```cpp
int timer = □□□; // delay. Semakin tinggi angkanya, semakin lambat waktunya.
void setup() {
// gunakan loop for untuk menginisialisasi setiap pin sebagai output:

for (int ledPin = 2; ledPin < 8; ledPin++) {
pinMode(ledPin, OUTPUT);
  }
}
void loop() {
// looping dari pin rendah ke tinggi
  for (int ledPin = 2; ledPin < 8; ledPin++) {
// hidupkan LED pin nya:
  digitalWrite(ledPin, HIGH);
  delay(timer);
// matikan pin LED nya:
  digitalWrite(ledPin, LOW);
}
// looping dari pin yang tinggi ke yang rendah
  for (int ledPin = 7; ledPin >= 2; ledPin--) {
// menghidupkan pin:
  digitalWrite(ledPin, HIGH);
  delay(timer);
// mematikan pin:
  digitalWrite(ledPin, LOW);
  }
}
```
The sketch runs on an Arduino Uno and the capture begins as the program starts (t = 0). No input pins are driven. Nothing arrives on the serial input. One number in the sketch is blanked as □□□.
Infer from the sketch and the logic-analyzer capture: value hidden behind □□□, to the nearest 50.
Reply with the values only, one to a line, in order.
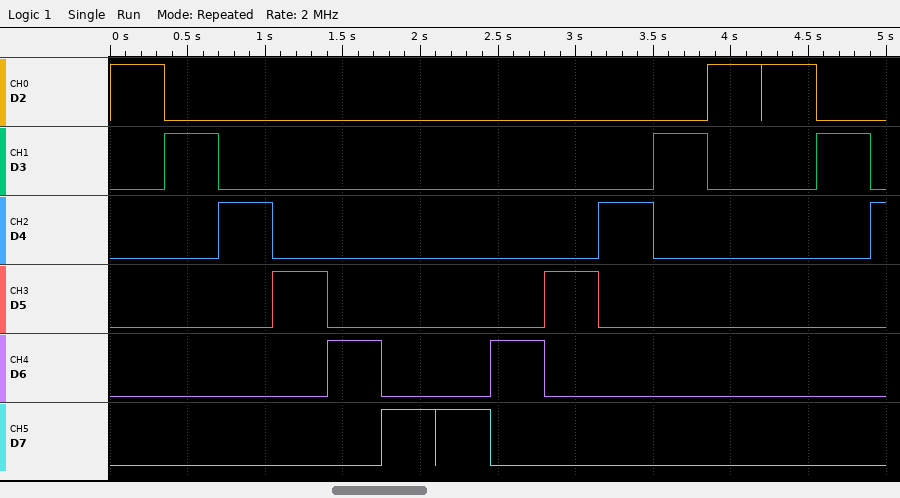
350
